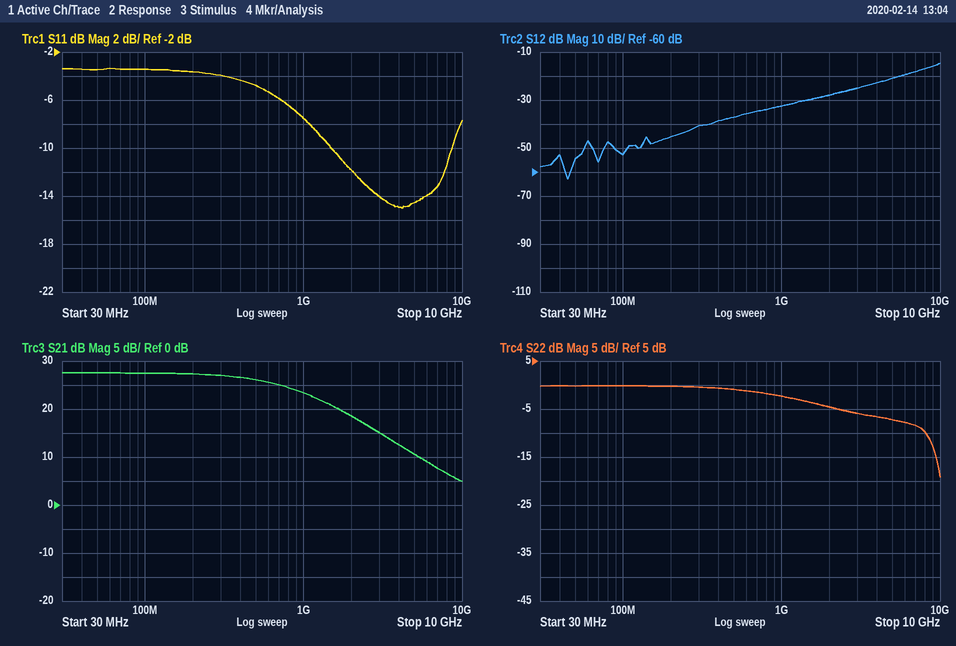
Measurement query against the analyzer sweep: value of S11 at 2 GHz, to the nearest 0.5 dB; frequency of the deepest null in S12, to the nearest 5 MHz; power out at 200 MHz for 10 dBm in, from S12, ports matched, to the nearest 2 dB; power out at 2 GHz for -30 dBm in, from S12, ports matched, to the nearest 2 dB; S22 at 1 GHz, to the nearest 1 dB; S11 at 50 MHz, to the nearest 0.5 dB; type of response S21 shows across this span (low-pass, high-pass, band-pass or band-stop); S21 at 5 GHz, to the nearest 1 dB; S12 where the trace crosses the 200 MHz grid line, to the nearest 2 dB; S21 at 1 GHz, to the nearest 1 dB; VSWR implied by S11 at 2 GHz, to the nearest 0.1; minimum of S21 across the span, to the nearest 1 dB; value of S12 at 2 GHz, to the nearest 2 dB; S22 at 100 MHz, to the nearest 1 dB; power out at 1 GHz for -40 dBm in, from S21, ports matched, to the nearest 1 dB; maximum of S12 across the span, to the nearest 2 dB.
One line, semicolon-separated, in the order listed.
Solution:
-12.0 dB; 45 MHz; -36 dBm; -58 dBm; -2 dB; -3.5 dB; low-pass; 11 dB; -46 dB; 23 dB; 1.7; 5 dB; -28 dB; 0 dB; -17 dBm; -14 dB
